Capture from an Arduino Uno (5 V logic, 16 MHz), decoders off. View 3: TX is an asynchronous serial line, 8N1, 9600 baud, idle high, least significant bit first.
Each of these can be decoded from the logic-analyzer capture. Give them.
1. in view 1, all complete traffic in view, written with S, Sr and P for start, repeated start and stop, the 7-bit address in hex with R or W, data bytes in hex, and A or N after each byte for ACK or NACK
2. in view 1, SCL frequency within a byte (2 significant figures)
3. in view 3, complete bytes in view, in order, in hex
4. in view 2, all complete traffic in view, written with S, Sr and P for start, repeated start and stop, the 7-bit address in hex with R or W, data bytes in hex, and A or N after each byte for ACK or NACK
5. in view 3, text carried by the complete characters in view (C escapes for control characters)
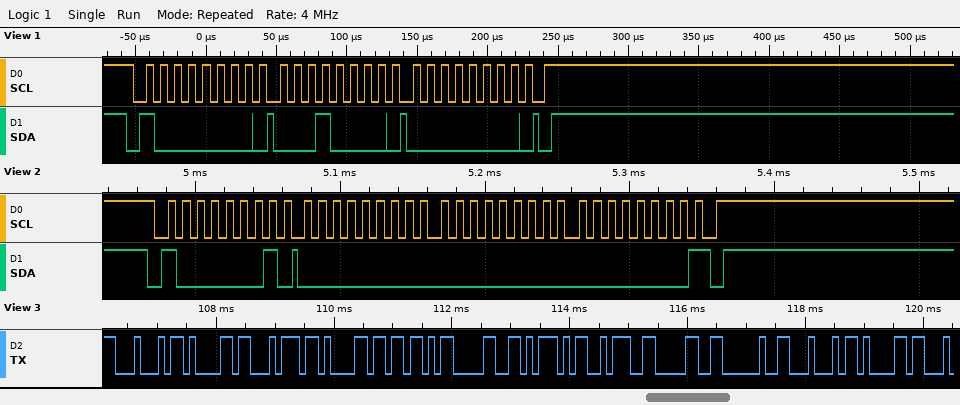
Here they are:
S 40W A 10 A 00 A P
100 kHz
44 61 74 61 5B 30 5D 3A 30 20 44 61
S 40R A 00 A 00 A 00 N P
"Data[0]:0 Da"
